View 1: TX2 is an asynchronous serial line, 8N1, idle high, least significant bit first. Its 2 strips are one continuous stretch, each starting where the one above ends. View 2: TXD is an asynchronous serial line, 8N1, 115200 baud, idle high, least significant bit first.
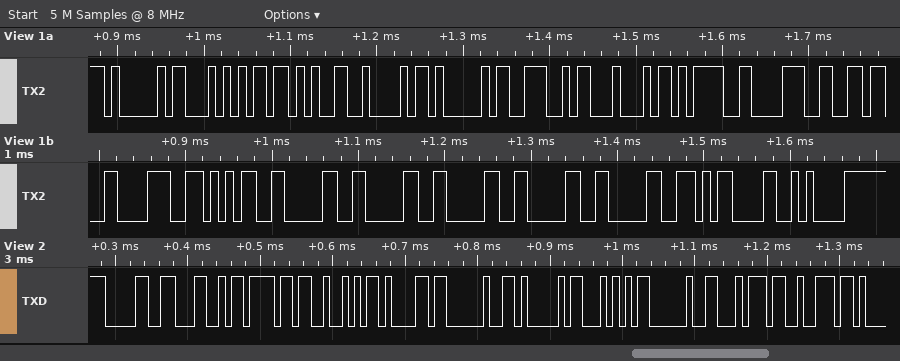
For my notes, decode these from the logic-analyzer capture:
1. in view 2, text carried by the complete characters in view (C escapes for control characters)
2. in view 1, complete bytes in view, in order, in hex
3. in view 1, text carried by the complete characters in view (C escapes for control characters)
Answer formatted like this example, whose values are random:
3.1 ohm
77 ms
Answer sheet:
"0LoRa AT tr"
41 54 2B 42 41 4E 44 3D 38 36 38 35 30 30 30 30 30 0D 0A
"AT+BAND=868500000\r\n"
